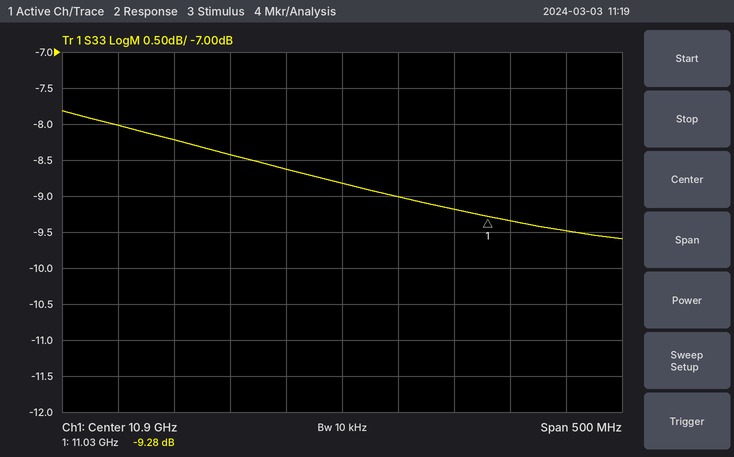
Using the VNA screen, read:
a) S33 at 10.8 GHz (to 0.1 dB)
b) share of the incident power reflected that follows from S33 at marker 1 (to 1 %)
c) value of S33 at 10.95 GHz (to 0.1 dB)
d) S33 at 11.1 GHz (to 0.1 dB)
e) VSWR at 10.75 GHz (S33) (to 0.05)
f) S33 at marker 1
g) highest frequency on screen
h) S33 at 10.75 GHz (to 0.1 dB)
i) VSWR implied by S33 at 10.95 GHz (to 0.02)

-8.4 dB
12 %
-9.0 dB
-9.5 dB
2.25
-9.28 dB
11.15 GHz
-8.2 dB
2.10
